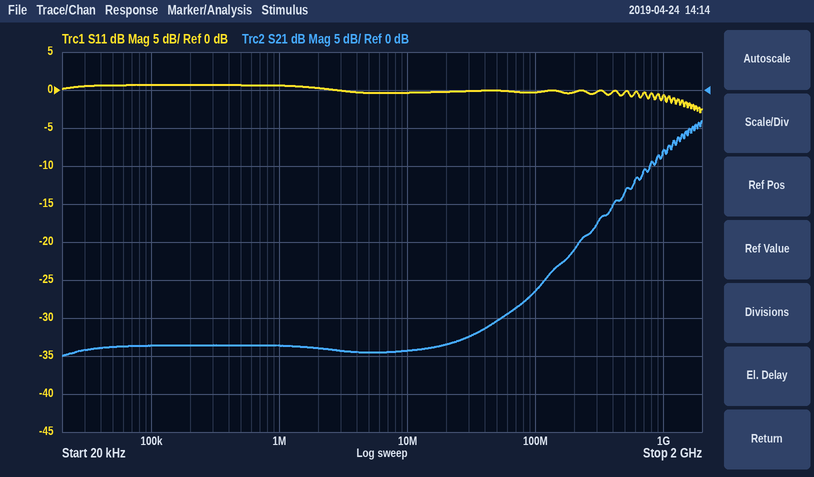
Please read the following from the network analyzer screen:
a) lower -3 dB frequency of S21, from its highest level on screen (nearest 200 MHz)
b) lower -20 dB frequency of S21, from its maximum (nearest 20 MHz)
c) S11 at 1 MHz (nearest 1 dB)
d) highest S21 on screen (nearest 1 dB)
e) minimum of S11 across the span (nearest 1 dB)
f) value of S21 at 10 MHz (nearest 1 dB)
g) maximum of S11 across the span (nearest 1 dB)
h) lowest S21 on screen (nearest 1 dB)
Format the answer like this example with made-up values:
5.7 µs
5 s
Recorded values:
1.2 GHz
140 MHz
1 dB
-4 dB
-3 dB
-34 dB
1 dB
-35 dB
